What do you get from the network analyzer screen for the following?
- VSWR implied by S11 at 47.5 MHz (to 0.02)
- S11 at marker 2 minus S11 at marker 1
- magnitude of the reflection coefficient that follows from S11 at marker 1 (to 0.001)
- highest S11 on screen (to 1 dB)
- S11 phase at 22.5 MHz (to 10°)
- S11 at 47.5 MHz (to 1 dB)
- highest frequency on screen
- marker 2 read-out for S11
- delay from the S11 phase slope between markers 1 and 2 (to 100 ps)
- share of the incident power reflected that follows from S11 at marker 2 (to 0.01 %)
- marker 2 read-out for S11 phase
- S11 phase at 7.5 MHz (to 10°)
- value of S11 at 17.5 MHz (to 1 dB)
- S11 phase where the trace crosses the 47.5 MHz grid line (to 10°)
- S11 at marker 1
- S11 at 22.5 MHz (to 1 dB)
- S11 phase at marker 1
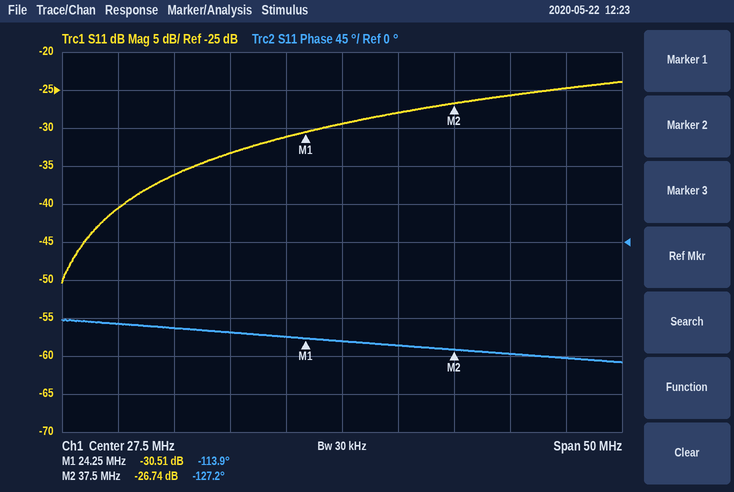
1.12
3.77 dB
0.030
-24 dB
-110°
-25 dB
52.5 MHz
-26.74 dB
2.8 ns
0.21 %
-127.2°
-100°
-33 dB
-140°
-30.51 dB
-31 dB
-113.9°
